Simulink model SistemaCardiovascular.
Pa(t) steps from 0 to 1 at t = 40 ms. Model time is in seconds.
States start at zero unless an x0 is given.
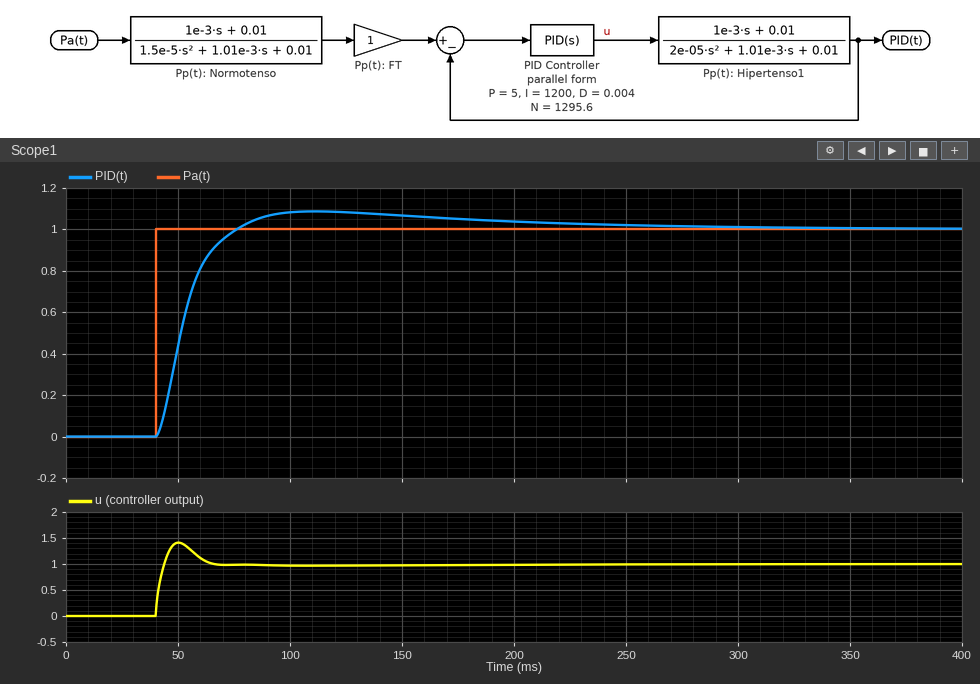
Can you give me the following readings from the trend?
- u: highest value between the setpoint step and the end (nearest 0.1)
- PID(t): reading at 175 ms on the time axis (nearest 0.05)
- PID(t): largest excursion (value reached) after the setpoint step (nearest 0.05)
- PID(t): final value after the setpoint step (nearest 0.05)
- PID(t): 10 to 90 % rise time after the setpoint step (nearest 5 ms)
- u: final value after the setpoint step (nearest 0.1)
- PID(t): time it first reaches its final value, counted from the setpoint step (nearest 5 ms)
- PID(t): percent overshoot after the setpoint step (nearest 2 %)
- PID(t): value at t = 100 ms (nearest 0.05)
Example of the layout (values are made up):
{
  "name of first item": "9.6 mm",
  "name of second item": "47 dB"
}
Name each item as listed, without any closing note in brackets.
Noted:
{
  "u: highest value between the setpoint step and the end": "1.4",
  "PID(t): reading at 175 ms on the time axis": "1.05",
  "PID(t): largest excursion (value reached) after the setpoint step": "1.10",
  "PID(t): final value after the setpoint step": "1.00",
  "PID(t): 10 to 90 % rise time after the setpoint step": "20 ms",
  "u: final value after the setpoint step": "1.0",
  "PID(t): time it first reaches its final value, counted from the setpoint step": "35 ms",
  "PID(t): percent overshoot after the setpoint step": "8 %",
  "PID(t): value at t = 100 ms": "1.10"
}
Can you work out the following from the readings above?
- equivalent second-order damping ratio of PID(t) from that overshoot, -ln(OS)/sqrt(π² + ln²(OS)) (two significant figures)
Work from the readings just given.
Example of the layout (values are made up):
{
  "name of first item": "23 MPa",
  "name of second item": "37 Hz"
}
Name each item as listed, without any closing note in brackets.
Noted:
{
  "equivalent second-order damping ratio of PID(t) from that overshoot, -ln(OS)/sqrt(π² + ln²(OS))": "0.63"
}
